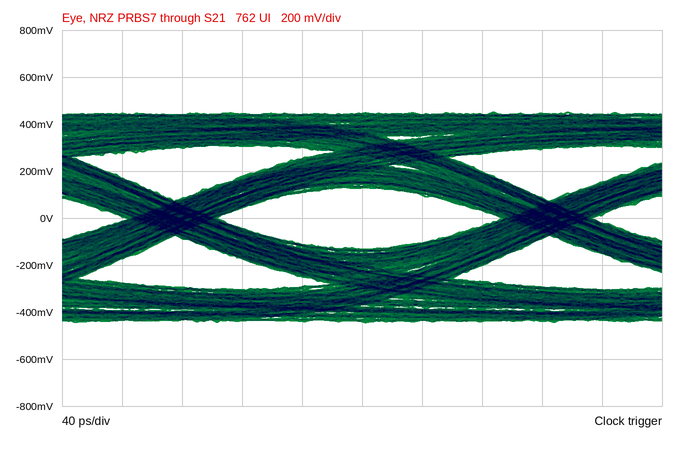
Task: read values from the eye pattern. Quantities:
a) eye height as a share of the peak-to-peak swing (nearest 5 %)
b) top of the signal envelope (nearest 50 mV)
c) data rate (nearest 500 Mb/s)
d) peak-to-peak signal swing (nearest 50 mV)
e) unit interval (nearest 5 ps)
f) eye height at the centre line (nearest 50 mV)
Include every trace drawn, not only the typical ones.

30 %
450 mV
4.0 Gb/s
900 mV
250 ps
250 mV
